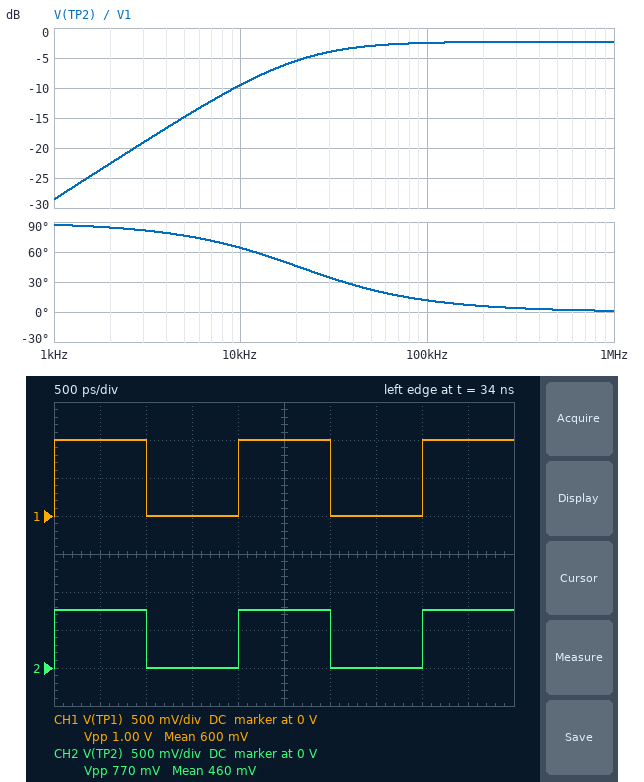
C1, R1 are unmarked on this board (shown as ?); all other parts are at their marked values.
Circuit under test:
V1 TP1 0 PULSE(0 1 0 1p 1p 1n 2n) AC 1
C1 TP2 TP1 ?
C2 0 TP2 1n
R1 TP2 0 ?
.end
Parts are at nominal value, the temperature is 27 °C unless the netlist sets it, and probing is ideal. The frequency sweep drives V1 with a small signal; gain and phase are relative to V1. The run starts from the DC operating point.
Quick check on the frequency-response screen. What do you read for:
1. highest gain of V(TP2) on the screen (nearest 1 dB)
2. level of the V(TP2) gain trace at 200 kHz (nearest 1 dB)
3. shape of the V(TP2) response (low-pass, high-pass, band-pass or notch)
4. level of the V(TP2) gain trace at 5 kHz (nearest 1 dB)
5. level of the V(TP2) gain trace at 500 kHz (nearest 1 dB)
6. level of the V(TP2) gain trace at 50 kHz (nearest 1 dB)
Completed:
-2 dB
-2 dB
high-pass
-15 dB
-2 dB
-3 dB
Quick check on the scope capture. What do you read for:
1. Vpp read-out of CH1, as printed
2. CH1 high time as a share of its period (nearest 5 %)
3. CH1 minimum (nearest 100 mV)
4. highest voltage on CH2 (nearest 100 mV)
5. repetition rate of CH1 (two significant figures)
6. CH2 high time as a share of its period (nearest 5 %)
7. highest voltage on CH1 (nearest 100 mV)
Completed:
1.00 V
50 %
0 V
800 mV
500 MHz
50 %
1.0 V
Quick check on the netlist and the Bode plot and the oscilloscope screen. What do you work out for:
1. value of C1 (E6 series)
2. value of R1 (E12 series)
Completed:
3.3 nF
1.8 kΩ
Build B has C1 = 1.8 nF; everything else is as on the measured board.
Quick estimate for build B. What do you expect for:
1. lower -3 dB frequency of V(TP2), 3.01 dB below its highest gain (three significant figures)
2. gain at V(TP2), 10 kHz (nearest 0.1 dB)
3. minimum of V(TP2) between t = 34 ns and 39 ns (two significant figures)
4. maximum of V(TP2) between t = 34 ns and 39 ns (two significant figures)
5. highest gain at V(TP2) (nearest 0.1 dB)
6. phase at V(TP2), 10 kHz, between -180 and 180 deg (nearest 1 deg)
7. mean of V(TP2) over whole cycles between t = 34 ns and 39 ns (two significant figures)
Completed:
31.6 kHz
-14.2 dB
-2.4 mV
640 mV
-3.8 dB
72 deg
320 mV
